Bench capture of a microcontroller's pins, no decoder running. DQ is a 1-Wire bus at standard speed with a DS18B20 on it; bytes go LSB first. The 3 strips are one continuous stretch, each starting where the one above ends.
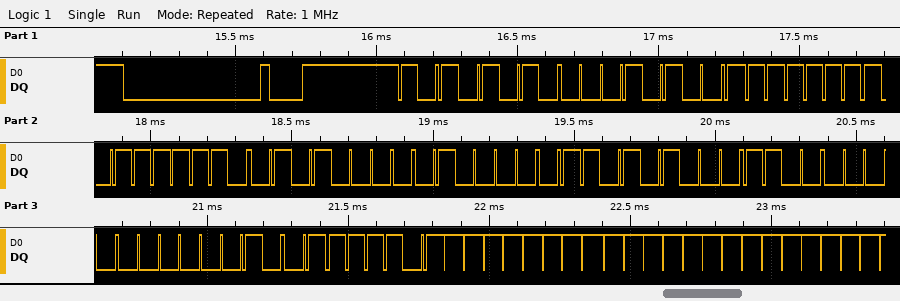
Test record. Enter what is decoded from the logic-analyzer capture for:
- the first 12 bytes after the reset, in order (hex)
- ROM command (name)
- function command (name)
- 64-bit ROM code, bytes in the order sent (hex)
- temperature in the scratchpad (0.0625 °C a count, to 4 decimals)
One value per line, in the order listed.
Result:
55 28 FF 7E 0A 82 15 03 40 BE FF FF
Match ROM
Read Scratchpad
28 FF 7E 0A 82 15 03 40
-0.0625 °C
